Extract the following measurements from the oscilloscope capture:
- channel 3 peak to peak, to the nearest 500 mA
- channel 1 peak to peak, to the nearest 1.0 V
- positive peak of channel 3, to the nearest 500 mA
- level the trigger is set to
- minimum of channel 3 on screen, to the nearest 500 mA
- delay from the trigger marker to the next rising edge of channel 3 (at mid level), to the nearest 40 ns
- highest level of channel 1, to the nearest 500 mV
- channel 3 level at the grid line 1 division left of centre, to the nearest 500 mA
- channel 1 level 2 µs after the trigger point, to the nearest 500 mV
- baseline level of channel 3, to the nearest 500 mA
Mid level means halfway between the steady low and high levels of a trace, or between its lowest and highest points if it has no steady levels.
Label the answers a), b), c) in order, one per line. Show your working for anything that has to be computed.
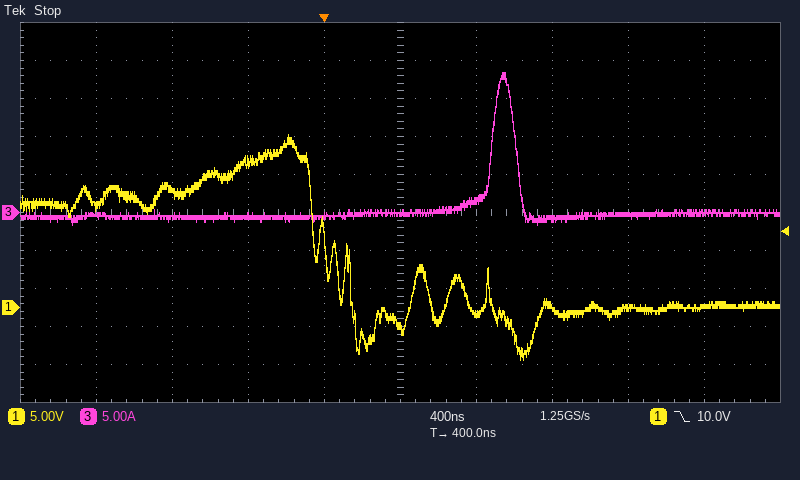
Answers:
a) 18.5 A − (-1.5 A) = 20.0 A
b) 30.0 V
c) 18.5 A
d) 10.0 V
e) -1.5 A
f) 880 ns
g) 23.0 V
h) -500 mA
i) 0.0 V
j) -500 mA
